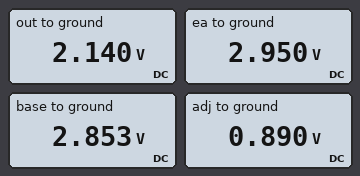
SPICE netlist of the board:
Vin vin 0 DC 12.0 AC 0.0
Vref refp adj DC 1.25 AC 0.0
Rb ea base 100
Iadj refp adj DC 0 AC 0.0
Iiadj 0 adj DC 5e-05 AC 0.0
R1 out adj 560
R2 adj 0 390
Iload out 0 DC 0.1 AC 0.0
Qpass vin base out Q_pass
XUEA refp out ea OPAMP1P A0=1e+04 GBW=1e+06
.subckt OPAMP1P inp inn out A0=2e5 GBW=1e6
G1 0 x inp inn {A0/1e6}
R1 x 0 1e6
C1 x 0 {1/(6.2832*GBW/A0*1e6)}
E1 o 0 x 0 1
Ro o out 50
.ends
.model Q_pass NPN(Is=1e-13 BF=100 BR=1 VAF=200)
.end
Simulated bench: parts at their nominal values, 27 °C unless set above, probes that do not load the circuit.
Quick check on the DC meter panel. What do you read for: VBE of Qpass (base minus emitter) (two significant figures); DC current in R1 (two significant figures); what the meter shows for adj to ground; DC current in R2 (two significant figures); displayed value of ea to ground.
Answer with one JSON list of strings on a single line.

["710 mV", "2.2 mA", "0.890 V", "2.3 mA", "2.950 V"]
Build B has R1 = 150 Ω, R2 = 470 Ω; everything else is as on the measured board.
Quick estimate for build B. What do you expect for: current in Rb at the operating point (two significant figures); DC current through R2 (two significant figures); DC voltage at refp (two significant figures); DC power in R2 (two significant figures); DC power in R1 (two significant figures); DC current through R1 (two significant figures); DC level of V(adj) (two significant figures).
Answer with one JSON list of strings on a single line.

["1.0 mA", "8.4 mA", "5.2 V", "33 mW", "10 mW", "8.3 mA", "3.9 V"]
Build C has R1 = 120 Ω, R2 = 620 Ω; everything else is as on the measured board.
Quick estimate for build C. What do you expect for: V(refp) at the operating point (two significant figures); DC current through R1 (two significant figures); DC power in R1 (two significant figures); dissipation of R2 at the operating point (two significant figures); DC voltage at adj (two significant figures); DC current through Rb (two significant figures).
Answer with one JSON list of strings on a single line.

["7.7 V", "10 mA", "13 mW", "68 mW", "6.5 V", "1.1 mA"]
